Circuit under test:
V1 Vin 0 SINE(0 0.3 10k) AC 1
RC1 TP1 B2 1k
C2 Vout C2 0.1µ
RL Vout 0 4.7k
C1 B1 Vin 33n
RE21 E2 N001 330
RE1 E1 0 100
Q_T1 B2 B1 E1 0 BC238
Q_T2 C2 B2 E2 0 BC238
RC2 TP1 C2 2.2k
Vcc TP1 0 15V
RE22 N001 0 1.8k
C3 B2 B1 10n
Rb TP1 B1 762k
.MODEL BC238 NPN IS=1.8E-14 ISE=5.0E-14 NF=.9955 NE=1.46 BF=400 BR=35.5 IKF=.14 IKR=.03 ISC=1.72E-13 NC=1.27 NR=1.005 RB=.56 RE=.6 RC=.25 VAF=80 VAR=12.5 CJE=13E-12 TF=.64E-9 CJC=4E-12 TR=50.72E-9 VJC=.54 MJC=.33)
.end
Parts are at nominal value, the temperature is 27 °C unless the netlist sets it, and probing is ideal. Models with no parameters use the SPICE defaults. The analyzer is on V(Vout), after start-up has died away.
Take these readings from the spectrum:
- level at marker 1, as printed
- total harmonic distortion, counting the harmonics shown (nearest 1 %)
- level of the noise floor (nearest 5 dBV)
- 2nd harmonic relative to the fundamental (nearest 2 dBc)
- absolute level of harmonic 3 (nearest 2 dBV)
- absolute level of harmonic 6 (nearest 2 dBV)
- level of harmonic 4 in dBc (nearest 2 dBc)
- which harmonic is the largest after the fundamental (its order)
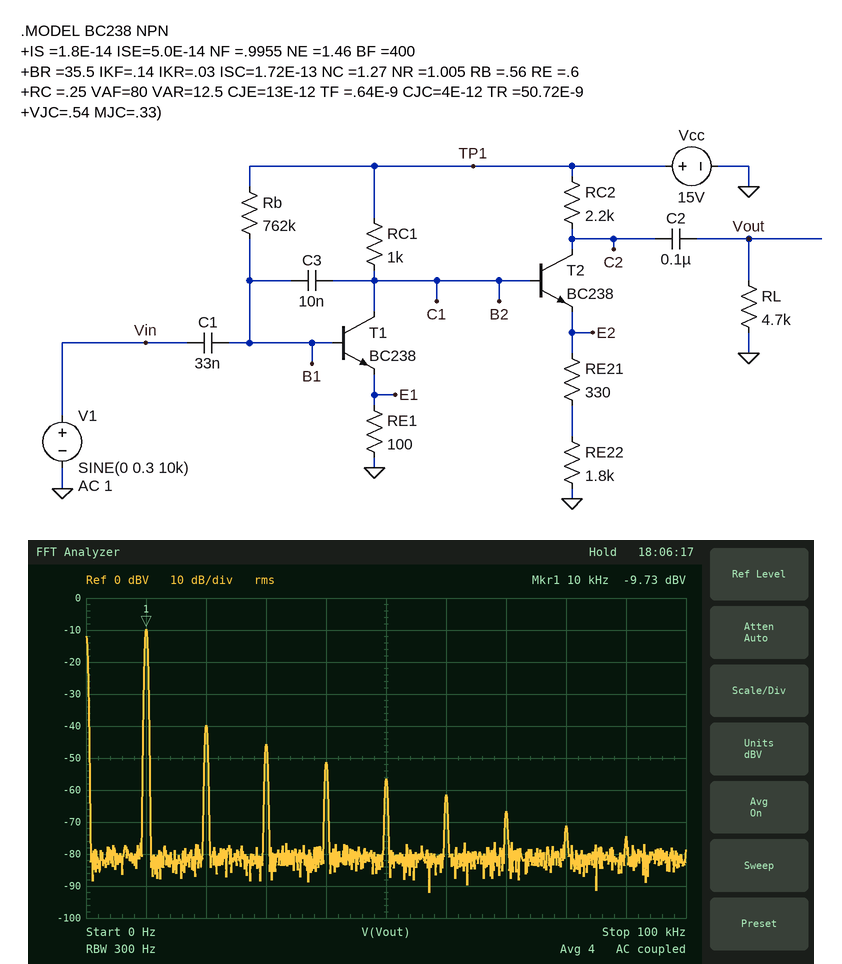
-9.73 dBV
4 %
-80 dBV
-30 dBc
-46 dBV
-62 dBV
-42 dBc
2
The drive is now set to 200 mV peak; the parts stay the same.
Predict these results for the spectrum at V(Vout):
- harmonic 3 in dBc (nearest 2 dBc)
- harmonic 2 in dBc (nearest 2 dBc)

-50 dBc
-40 dBc
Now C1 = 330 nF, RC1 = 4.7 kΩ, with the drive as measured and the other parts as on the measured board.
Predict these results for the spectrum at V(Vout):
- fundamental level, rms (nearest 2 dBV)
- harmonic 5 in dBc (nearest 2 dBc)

4 dBV
-40 dBc
